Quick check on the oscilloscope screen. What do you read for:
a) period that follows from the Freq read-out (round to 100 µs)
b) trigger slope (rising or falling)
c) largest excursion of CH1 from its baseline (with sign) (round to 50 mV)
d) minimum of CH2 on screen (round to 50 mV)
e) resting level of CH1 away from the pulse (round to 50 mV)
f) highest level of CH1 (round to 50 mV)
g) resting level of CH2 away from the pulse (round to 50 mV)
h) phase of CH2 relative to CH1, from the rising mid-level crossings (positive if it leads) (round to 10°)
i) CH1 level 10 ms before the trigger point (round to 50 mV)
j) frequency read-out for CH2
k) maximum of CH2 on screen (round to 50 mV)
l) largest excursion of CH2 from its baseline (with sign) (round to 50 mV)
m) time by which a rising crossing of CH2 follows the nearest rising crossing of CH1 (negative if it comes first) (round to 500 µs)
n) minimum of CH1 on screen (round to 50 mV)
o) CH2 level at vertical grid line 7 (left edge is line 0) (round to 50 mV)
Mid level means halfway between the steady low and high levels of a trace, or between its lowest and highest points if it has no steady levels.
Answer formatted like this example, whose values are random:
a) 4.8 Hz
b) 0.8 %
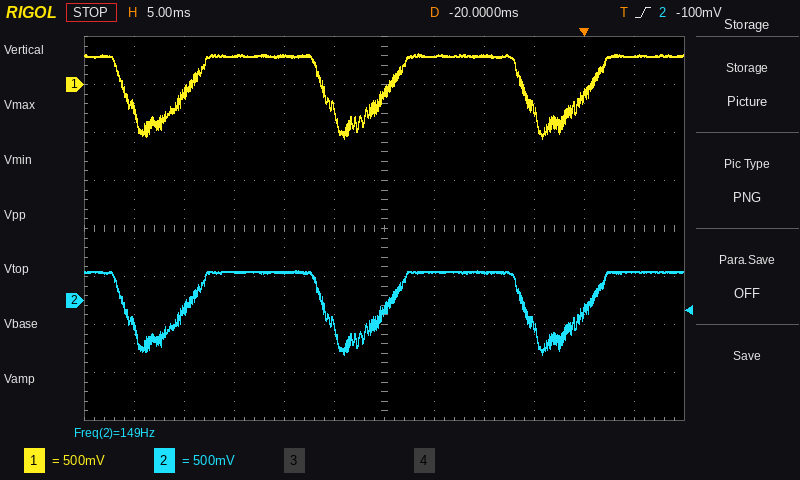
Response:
a) 6.7 ms
b) rising
c) -850 mV
d) -550 mV
e) 300 mV
f) 300 mV
g) 300 mV
h) 0°
i) 300 mV
j) 149 Hz
k) 300 mV
l) -850 mV
m) 0.0 ms
n) -550 mV
o) 300 mV
